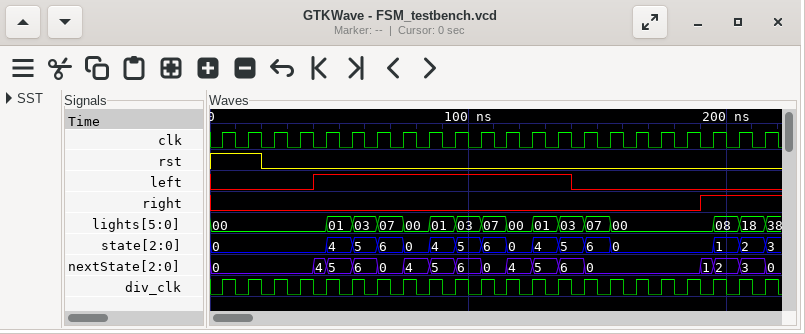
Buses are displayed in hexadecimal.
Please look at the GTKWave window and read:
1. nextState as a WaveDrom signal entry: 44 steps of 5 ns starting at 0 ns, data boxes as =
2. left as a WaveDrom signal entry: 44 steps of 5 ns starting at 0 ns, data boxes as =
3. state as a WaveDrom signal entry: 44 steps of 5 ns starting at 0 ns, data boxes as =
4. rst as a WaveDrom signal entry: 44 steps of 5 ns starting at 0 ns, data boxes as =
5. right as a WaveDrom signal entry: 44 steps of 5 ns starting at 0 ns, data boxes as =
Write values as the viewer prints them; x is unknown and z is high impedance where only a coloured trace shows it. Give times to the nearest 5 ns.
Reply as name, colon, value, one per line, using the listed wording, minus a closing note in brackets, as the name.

nextState as a WaveDrom signal entry: 44 steps of 5 ns starting at 0 ns, data boxes as =: {name: 'nextState', wave: '=.......==.=.=.=.=.=.=.=.=.=.=........==.=.=', data: '0 4 5 6 0 4 5 6 0 4 5 6 0 1 2 3 0'}
left as a WaveDrom signal entry: 44 steps of 5 ns starting at 0 ns, data boxes as =: {name: 'left', wave: '0.......1...................0...............'}
state as a WaveDrom signal entry: 44 steps of 5 ns starting at 0 ns, data boxes as =: {name: 'state', wave: '=........=.=.=.=.=.=.=.=.=.=.=.=.......=.=.=', data: '0 4 5 6 0 4 5 6 0 4 5 6 0 1 2 3'}
rst as a WaveDrom signal entry: 44 steps of 5 ns starting at 0 ns, data boxes as =: {name: 'rst', wave: '1...0.......................................'}
right as a WaveDrom signal entry: 44 steps of 5 ns starting at 0 ns, data boxes as =: {name: 'right', wave: '0.....................................1.....'}
